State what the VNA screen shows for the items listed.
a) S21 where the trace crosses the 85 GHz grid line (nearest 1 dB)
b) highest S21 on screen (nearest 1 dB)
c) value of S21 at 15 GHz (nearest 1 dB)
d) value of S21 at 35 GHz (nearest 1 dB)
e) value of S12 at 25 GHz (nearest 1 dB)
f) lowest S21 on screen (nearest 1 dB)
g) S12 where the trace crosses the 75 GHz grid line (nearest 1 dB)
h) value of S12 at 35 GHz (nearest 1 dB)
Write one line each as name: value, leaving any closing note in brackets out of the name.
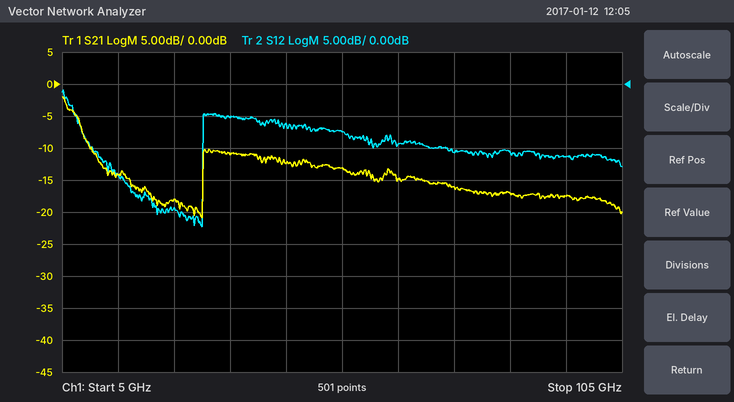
S21 where the trace crosses the 85 GHz grid line: -17 dB
highest S21 on screen: -2 dB
value of S21 at 15 GHz: -14 dB
value of S21 at 35 GHz: -11 dB
value of S12 at 25 GHz: -19 dB
lowest S21 on screen: -21 dB
S12 where the trace crosses the 75 GHz grid line: -11 dB
value of S12 at 35 GHz: -5 dB
